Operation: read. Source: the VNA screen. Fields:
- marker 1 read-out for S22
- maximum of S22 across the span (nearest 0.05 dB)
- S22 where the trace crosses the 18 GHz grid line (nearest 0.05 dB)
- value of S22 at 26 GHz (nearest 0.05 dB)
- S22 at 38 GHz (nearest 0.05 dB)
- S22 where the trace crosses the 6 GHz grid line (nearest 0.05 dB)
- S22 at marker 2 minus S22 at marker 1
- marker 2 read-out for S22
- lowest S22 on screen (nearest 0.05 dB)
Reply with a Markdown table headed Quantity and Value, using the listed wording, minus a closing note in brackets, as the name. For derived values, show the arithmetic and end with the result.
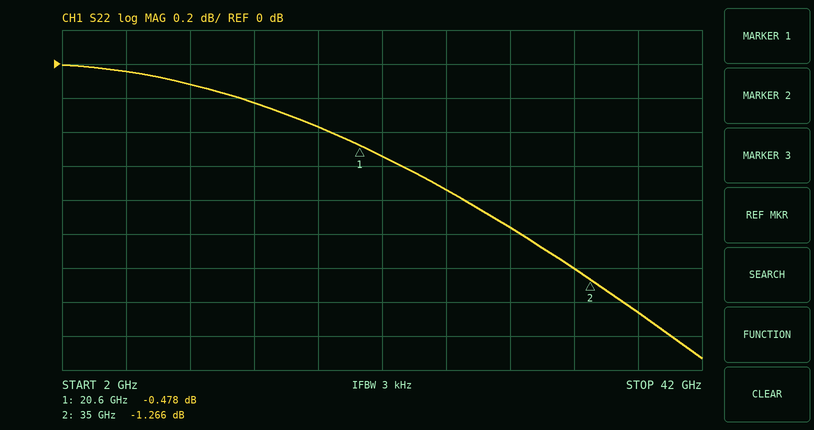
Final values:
| Quantity | Value |
|---|---|
| marker 1 read-out for S22 | -0.478 dB |
| maximum of S22 across the span | 0.00 dB |
| S22 where the trace crosses the 18 GHz grid line | -0.35 dB |
| value of S22 at 26 GHz | -0.75 dB |
| S22 at 38 GHz | -1.45 dB |
| S22 where the trace crosses the 6 GHz grid line | -0.05 dB |
| S22 at marker 2 minus S22 at marker 1 | -1.266 − (-0.478) = -0.788 dB |
| marker 2 read-out for S22 | -1.266 dB |
| lowest S22 on screen | -1.75 dB |
